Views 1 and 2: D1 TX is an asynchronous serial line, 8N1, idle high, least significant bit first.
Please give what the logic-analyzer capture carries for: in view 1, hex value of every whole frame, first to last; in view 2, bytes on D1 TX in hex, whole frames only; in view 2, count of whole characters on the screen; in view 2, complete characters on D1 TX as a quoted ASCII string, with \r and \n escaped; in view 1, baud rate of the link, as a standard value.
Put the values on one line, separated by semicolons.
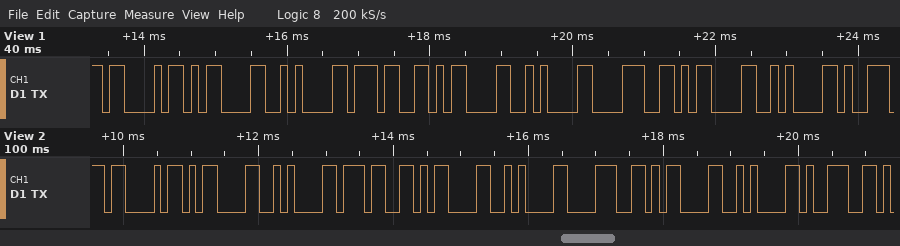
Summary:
43 0D 0A 37 0D 0A 38 0D 0A; 43 0D 0A 37 0D 0A 38 0D 0A 39; 10; "C\r\n7\r\n8\r\n9"; 9600 baud
